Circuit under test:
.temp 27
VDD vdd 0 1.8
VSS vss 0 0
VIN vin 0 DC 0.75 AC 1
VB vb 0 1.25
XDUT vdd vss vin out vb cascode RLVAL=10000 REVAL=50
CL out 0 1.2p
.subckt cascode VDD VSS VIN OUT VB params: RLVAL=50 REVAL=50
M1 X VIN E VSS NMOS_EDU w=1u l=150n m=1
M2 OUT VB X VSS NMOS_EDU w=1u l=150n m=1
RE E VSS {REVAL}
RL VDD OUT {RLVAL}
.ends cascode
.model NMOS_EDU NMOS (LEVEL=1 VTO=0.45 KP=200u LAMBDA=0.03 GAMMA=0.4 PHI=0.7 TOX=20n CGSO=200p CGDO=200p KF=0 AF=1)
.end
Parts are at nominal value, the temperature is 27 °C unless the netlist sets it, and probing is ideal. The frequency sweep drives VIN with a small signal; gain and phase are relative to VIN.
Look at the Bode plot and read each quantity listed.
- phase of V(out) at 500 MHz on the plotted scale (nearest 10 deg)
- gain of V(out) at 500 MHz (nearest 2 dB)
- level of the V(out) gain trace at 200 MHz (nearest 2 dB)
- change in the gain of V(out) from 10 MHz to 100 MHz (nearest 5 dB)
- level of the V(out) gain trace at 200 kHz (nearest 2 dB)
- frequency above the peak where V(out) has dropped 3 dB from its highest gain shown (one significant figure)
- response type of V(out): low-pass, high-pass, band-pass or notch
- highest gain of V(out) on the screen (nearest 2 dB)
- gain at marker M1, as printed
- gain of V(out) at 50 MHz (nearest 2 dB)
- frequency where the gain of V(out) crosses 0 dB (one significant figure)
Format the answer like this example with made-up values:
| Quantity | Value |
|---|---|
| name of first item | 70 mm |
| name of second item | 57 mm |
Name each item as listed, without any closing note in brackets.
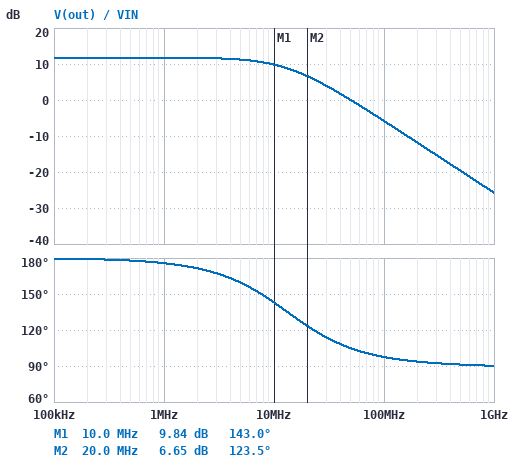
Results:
| Quantity | Value |
|---|---|
| phase of V(out) at 500 MHz on the plotted scale | 90 deg |
| gain of V(out) at 500 MHz | -20 dB |
| level of the V(out) gain trace at 200 MHz | -12 dB |
| change in the gain of V(out) from 10 MHz to 100 MHz | -15 dB |
| level of the V(out) gain trace at 200 kHz | 12 dB |
| frequency above the peak where V(out) has dropped 3 dB from its highest gain shown | 10 MHz |
| response type of V(out): low-pass, high-pass, band-pass or notch | low-pass |
| highest gain of V(out) on the screen | 12 dB |
| gain at marker M1, as printed | 9.84 dB |
| gain of V(out) at 50 MHz | 0 dB |
| frequency where the gain of V(out) crosses 0 dB | 50 MHz |
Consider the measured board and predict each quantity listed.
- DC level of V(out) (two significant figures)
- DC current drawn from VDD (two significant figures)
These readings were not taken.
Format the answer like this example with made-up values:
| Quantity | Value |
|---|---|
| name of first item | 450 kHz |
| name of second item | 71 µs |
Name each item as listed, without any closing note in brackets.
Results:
| Quantity | Value |
|---|---|
| DC level of V(out) | 1.2 V |
| DC current drawn from VDD | 59 µA |
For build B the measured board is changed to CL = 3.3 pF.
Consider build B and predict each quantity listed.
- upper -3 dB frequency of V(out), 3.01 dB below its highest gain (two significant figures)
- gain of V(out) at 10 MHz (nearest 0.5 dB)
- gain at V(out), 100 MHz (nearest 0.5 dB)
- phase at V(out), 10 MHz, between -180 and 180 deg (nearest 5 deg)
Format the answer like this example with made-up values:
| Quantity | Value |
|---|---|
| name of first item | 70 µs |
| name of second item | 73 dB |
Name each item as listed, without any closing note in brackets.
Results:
| Quantity | Value |
|---|---|
| upper -3 dB frequency of V(out), 3.01 dB below its highest gain | 4.8 MHz |
| gain of V(out) at 10 MHz | 4.5 dB |
| gain at V(out), 100 MHz | -14.5 dB |
| phase at V(out), 10 MHz, between -180 and 180 deg | 115 deg |
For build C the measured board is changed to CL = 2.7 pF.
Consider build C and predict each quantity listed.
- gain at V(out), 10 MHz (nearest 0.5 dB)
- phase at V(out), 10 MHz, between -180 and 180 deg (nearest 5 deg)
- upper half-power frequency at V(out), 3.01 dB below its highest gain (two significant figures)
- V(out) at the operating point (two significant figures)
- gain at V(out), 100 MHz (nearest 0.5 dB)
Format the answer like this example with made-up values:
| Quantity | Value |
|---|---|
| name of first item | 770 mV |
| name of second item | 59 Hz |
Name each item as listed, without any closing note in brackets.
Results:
| Quantity | Value |
|---|---|
| gain at V(out), 10 MHz | 6.0 dB |
| phase at V(out), 10 MHz, between -180 and 180 deg | 120 deg |
| upper half-power frequency at V(out), 3.01 dB below its highest gain | 5.9 MHz |
| V(out) at the operating point | 1.2 V |
| gain at V(out), 100 MHz | -13.0 dB |
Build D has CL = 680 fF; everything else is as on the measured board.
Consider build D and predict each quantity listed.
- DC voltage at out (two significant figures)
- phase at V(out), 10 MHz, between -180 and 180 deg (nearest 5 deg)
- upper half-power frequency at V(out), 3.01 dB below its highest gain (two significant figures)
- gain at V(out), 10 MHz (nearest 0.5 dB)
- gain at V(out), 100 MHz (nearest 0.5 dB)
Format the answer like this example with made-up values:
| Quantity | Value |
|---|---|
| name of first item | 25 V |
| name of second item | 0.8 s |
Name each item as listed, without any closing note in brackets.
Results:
| Quantity | Value |
|---|---|
| DC voltage at out | 1.2 V |
| phase at V(out), 10 MHz, between -180 and 180 deg | 155 deg |
| upper half-power frequency at V(out), 3.01 dB below its highest gain | 23 MHz |
| gain at V(out), 10 MHz | 11.0 dB |
| gain at V(out), 100 MHz | -1.0 dB |
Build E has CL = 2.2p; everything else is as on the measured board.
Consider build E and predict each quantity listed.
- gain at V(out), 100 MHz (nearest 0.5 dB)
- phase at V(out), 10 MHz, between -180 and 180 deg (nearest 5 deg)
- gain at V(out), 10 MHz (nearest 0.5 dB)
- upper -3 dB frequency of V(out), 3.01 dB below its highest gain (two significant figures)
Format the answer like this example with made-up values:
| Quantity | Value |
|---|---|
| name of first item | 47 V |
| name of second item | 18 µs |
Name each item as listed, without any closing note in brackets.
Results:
| Quantity | Value |
|---|---|
| gain at V(out), 100 MHz | -11.0 dB |
| phase at V(out), 10 MHz, between -180 and 180 deg | 125 deg |
| gain at V(out), 10 MHz | 7.0 dB |
| upper -3 dB frequency of V(out), 3.01 dB below its highest gain | 7.2 MHz |
